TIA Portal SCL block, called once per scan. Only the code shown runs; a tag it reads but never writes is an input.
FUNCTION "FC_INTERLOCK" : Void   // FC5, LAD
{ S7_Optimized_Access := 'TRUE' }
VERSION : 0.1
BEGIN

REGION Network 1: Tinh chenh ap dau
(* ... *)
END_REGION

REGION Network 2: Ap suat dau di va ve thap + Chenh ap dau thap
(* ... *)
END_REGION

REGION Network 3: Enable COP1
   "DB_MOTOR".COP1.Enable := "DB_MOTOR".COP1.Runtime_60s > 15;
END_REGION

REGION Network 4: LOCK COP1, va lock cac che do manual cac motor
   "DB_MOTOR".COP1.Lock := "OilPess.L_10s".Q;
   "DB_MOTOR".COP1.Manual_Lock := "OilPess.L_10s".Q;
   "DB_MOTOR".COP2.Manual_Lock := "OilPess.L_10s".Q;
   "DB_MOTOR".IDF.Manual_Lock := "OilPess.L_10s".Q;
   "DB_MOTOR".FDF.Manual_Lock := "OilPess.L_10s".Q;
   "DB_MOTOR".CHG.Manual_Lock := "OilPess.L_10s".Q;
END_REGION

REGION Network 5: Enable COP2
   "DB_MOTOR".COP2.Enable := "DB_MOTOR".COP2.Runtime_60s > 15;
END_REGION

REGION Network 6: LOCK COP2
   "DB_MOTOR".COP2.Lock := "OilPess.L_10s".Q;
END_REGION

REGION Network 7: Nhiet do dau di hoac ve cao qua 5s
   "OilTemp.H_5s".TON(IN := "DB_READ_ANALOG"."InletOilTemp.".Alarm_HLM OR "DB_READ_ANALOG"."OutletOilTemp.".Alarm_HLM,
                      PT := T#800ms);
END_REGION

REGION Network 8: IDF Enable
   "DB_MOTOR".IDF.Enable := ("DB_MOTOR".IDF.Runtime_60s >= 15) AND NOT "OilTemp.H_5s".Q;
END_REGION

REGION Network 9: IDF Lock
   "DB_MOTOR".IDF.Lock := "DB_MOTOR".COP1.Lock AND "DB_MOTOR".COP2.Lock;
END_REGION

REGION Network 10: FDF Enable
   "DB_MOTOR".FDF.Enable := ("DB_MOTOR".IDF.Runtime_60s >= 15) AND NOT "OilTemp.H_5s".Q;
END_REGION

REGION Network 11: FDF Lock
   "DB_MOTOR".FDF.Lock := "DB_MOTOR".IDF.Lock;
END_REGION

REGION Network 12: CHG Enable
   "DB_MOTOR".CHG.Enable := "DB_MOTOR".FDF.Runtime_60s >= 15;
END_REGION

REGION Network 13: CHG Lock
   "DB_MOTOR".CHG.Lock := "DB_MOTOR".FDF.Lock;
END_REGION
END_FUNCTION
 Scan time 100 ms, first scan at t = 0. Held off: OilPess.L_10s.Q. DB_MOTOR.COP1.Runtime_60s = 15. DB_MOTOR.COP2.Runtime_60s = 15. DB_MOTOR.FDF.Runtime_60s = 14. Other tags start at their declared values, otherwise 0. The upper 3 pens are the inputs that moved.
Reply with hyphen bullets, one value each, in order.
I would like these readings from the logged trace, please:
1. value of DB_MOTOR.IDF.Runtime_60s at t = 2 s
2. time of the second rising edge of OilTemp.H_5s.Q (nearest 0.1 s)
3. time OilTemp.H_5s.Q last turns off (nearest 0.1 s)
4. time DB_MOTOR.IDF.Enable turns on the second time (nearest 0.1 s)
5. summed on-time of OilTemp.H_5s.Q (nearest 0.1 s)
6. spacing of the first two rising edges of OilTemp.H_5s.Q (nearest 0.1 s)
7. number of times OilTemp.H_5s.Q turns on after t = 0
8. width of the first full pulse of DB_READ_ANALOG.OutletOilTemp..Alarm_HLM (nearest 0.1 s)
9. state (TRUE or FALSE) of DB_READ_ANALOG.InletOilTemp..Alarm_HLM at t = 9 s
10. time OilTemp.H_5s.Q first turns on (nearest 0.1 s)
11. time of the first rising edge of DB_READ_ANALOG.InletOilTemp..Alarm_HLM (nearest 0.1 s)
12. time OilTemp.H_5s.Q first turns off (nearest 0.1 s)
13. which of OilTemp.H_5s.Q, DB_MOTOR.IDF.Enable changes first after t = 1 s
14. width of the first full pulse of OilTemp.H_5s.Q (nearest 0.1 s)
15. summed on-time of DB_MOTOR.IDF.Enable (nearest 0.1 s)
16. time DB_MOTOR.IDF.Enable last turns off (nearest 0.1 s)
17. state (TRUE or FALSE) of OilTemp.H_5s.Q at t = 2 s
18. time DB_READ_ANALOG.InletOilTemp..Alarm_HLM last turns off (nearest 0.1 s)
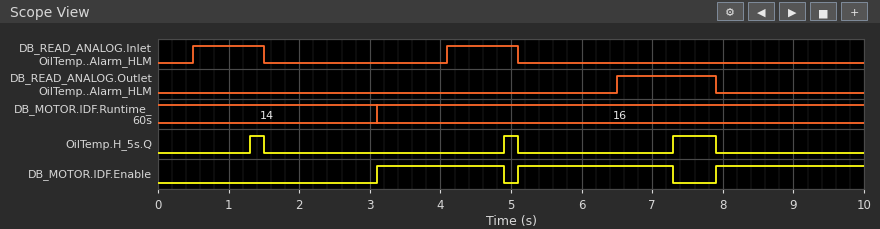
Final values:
- 14
- 4.9 s
- 7.9 s
- 5.1 s
- 1.0 s
- 3.6 s
- 3
- 1.4 s
- FALSE
- 1.3 s
- 0.5 s
- 1.5 s
- OilTemp.H_5s.Q
- 0.2 s
- 6.1 s
- 7.3 s
- FALSE
- 5.1 s
